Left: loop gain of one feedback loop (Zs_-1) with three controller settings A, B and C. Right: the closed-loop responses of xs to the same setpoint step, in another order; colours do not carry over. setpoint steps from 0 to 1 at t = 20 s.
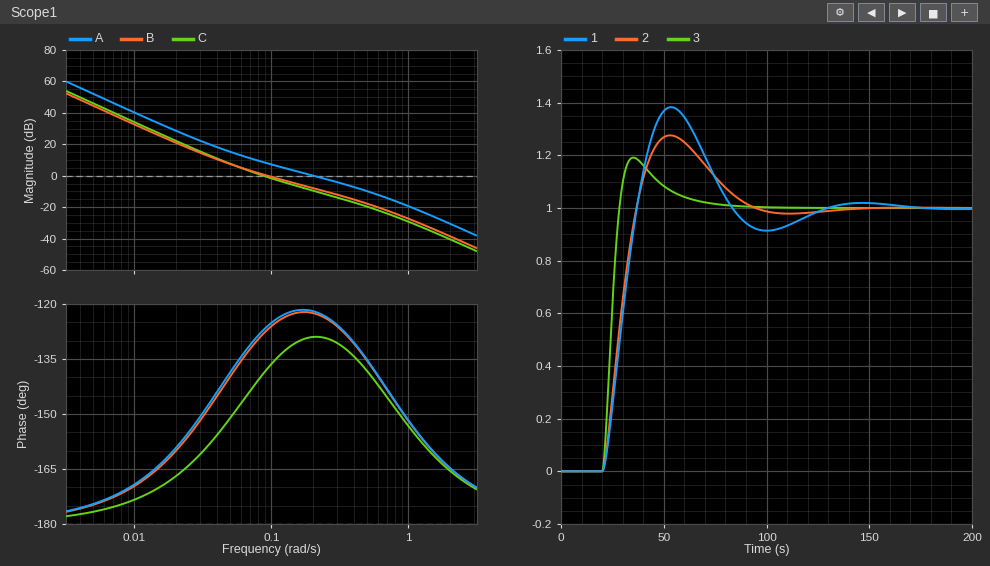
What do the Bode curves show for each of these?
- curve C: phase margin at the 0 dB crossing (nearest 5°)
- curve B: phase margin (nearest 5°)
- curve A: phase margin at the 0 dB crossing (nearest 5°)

40°
55°
60°
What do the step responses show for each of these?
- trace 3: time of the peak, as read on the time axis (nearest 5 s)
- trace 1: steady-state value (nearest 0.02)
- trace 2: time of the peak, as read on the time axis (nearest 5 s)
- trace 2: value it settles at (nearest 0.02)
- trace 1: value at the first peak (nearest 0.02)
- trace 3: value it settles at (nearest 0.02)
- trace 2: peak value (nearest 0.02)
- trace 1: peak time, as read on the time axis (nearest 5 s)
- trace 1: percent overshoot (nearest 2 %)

35 s
1.00
55 s
1.00
1.38
1.00
1.28
55 s
38 %
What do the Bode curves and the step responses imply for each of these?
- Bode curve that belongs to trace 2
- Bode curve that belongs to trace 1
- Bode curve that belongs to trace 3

B
C
A
